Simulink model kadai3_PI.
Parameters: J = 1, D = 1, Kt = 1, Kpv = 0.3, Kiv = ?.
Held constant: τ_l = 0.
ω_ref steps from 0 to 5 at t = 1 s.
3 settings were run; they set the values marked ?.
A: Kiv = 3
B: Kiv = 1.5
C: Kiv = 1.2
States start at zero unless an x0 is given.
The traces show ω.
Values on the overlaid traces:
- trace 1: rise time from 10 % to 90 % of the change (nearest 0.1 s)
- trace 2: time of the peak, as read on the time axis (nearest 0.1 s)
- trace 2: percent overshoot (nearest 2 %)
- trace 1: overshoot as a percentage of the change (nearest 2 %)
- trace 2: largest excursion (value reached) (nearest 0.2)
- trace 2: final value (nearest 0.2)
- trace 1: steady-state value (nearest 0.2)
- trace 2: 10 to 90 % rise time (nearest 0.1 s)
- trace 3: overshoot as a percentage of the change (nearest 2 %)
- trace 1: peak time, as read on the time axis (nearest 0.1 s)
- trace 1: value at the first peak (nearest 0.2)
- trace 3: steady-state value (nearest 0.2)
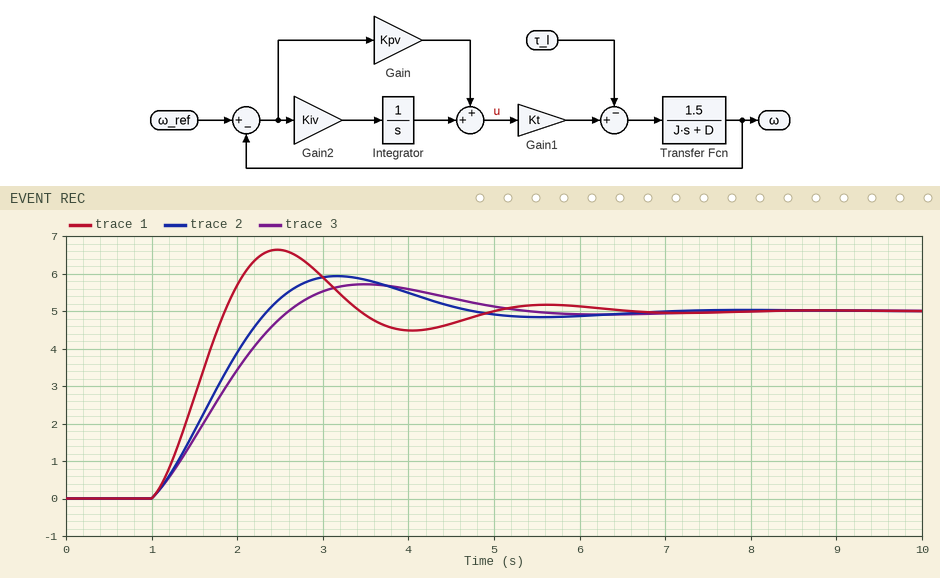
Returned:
0.6 s
3.2 s
18 %
32 %
6.0
5.0
5.0
1.0 s
14 %
2.5 s
6.6
5.0
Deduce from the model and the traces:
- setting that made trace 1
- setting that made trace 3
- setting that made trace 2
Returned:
A
C
B
